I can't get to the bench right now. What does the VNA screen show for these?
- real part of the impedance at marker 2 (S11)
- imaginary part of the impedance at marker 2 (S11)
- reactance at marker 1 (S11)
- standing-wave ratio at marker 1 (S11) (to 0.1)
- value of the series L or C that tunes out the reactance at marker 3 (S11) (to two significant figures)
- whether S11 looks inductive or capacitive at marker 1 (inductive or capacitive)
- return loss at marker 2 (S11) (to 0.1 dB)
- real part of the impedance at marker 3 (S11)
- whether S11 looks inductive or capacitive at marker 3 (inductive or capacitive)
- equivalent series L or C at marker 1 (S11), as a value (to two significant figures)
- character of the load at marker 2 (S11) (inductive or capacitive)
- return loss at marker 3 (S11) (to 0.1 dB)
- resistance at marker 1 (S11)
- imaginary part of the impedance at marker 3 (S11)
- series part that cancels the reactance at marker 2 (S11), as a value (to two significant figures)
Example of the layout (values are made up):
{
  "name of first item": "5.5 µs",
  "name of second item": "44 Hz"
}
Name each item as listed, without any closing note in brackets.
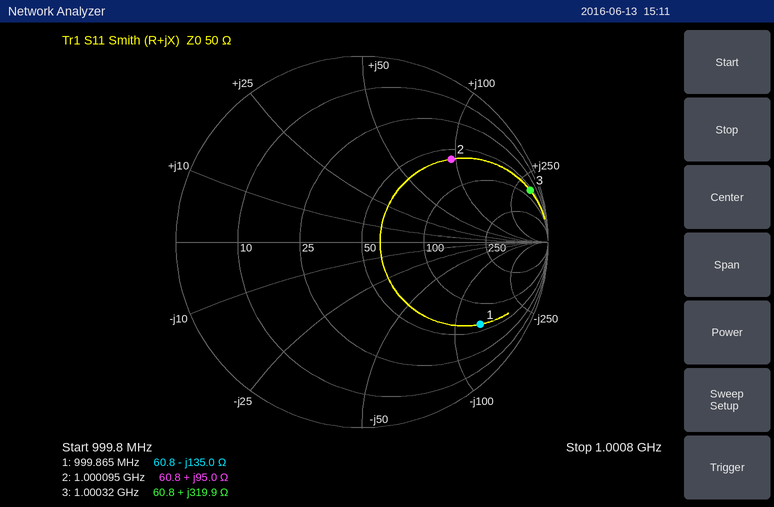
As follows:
{
  "real part of the impedance at marker 2": "60.8 Ω",
  "imaginary part of the impedance at marker 2": "+95.0 Ω",
  "reactance at marker 1": "-135.0 Ω",
  "standing-wave ratio at marker 1 (S11)": "7.9",
  "value of the series L or C that tunes out the reactance at marker 3 (S11)": "500 fF",
  "whether S11 looks inductive or capacitive at marker 1": "capacitive",
  "return loss at marker 2 (S11)": "3.7 dB",
  "real part of the impedance at marker 3": "60.8 Ω",
  "whether S11 looks inductive or capacitive at marker 3": "inductive",
  "equivalent series L or C at marker 1 (S11), as a value": "1.2 pF",
  "character of the load at marker 2 (S11)": "inductive",
  "return loss at marker 3 (S11)": "0.5 dB",
  "resistance at marker 1": "60.8 Ω",
  "imaginary part of the impedance at marker 3": "+319.9 Ω",
  "series part that cancels the reactance at marker 2 (S11), as a value": "1.7 pF"
}
